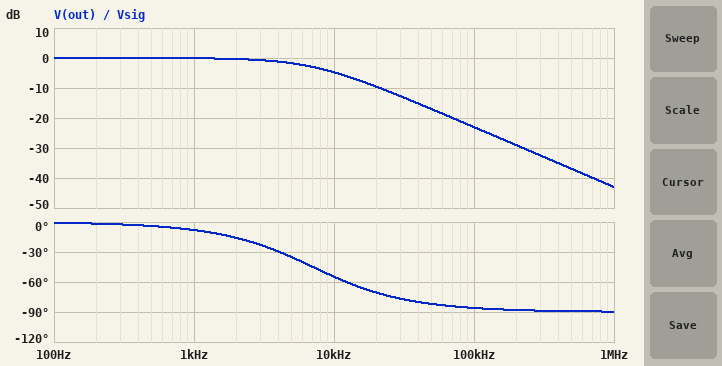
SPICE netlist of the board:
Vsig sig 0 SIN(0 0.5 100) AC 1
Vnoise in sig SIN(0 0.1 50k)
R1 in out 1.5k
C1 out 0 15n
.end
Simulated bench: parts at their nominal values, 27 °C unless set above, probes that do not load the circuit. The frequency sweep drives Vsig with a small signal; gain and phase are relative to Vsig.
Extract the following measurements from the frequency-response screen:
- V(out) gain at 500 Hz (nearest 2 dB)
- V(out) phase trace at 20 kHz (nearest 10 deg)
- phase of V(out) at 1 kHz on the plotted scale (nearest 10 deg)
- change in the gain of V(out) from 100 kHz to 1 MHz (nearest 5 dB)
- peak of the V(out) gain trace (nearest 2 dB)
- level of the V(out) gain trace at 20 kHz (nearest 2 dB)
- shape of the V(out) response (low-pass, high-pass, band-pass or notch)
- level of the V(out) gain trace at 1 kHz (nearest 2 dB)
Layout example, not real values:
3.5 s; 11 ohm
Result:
0 dB; -70 deg; -10 deg; -20 dB; 0 dB; -10 dB; low-pass; 0 dB
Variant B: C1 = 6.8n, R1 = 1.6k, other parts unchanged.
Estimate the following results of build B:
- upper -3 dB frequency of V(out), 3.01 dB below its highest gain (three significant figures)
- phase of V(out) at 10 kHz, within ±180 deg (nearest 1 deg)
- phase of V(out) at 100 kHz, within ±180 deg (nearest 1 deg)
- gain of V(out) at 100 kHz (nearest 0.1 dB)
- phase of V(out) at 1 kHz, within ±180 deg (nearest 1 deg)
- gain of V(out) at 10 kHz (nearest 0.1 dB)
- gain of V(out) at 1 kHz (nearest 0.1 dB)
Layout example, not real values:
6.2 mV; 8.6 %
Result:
14.6 kHz; -34 deg; -82 deg; -16.8 dB; -4 deg; -1.7 dB; 0 dB
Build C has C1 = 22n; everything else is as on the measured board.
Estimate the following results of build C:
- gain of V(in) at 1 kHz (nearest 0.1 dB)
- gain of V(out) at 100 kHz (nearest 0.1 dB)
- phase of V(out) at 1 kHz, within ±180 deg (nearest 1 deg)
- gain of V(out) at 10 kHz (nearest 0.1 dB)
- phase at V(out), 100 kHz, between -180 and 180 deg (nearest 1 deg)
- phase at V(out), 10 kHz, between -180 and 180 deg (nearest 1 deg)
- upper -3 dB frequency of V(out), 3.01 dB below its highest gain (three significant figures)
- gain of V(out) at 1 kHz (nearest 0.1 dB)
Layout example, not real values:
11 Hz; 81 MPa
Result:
0 dB; -26.3 dB; -12 deg; -7.2 dB; -87 deg; -64 deg; 4.82 kHz; -0.2 dB
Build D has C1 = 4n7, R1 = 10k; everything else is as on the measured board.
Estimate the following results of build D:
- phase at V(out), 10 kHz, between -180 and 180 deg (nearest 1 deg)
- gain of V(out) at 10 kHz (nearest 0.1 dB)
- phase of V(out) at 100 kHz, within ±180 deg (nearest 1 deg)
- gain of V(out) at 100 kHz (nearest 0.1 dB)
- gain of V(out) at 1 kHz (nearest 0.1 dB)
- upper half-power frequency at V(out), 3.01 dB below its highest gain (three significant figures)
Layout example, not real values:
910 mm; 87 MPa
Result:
-71 deg; -9.9 dB; -88 deg; -29.4 dB; -0.4 dB; 3.39 kHz
